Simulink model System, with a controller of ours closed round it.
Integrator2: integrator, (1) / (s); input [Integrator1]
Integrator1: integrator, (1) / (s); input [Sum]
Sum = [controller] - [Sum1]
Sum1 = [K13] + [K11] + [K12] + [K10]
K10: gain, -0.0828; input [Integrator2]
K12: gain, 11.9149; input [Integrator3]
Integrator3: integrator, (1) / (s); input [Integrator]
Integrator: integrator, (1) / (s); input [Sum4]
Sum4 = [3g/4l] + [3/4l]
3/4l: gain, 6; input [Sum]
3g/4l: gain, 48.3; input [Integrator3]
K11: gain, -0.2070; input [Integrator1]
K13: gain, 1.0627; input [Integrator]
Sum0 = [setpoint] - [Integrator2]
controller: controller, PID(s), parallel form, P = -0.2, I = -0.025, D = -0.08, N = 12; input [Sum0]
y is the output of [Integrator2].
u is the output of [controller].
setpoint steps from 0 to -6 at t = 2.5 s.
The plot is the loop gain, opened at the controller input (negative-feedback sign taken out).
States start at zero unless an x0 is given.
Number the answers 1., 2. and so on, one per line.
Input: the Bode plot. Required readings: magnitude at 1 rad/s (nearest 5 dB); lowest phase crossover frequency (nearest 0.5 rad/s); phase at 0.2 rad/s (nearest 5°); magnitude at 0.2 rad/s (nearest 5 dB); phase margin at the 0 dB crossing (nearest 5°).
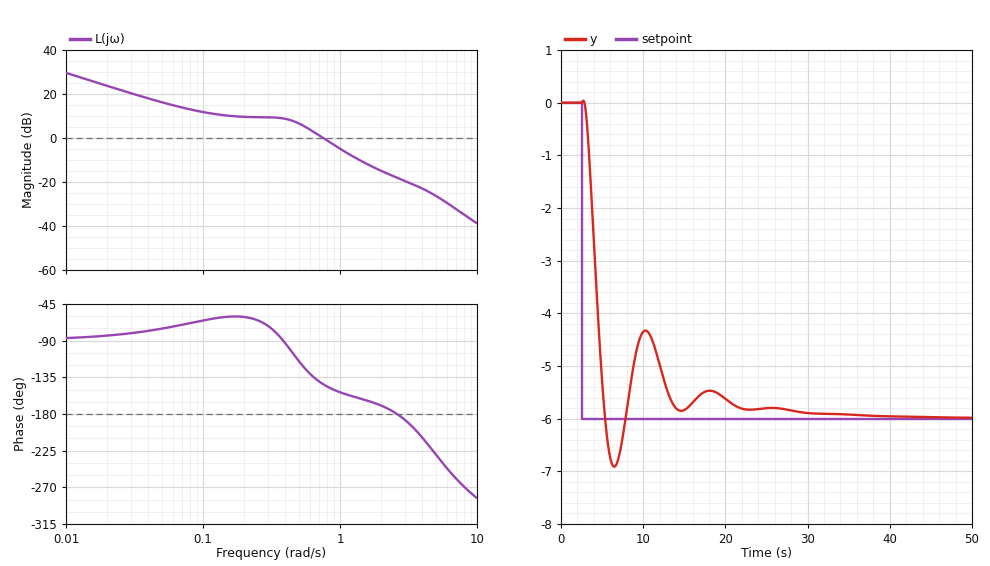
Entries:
1. -5 dB
2. 2.5 rad/s
3. -60°
4. 10 dB
5. 35°
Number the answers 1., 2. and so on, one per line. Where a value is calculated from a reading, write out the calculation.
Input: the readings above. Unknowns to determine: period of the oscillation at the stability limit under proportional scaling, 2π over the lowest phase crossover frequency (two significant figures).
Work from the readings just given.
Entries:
1. 2π / 2.5 = 2.5 s
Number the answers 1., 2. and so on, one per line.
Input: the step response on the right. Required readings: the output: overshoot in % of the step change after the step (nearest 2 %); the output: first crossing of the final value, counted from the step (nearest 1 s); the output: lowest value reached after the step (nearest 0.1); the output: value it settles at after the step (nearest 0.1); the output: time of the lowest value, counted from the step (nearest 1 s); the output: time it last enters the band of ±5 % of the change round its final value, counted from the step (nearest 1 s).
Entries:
1. 16 %
2. 3 s
3. -6.9
4. -6.0
5. 4 s
6. 18 s
